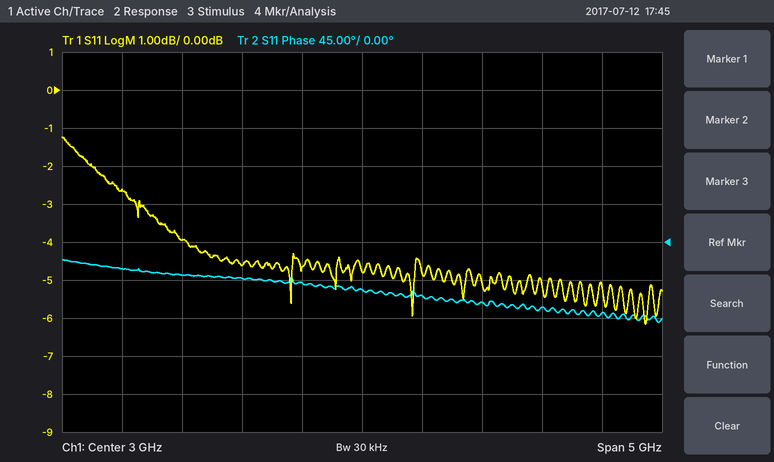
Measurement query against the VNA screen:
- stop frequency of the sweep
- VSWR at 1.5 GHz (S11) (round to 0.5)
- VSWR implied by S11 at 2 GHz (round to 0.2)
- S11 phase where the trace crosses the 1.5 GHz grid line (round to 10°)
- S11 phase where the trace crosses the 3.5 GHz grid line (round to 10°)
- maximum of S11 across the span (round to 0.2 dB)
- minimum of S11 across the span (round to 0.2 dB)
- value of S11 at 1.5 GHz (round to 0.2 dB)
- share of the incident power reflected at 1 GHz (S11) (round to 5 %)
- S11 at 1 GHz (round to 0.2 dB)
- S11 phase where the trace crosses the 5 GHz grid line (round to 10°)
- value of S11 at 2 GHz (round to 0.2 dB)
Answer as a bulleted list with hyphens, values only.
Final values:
- 5.5 GHz
- 4.5
- 3.8
- -40°
- -60°
- -1.2 dB
- -6.2 dB
- -4.0 dB
- 55 %
- -2.6 dB
- -80°
- -4.6 dB
